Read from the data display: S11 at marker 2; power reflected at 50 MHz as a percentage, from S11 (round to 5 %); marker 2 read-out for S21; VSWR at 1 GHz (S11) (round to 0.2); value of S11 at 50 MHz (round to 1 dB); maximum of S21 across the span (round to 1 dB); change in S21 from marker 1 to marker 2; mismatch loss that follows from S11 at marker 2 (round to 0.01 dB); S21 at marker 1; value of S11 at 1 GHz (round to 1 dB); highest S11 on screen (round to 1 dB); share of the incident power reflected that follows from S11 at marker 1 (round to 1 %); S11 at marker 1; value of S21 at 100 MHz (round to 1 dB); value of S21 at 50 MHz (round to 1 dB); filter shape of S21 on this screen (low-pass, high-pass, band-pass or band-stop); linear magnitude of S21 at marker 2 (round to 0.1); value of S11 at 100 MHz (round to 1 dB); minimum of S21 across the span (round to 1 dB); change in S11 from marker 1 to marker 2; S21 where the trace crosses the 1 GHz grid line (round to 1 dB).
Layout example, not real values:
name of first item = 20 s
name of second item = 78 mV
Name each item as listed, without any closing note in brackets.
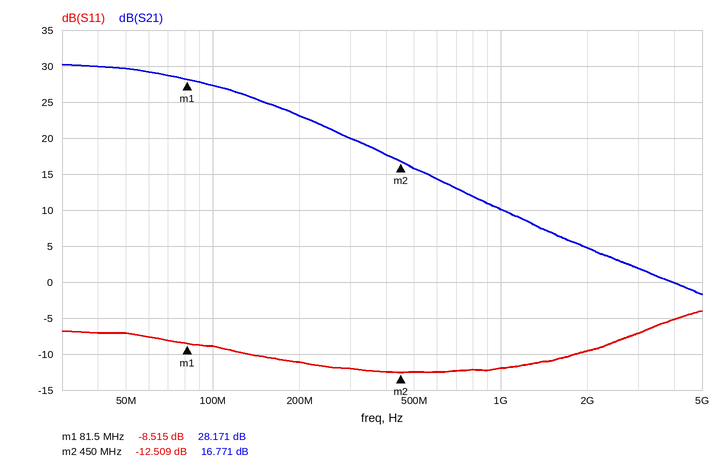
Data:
S11 at marker 2 = -12.509 dB
power reflected at 50 MHz as a percentage, from S11 = 20 %
marker 2 read-out for S21 = 16.771 dB
VSWR at 1 GHz (S11) = 1.6
value of S11 at 50 MHz = -7 dB
maximum of S21 across the span = 30 dB
change in S21 from marker 1 to marker 2 = -11.400 dB
mismatch loss that follows from S11 at marker 2 = 0.25 dB
S21 at marker 1 = 28.171 dB
value of S11 at 1 GHz = -12 dB
highest S11 on screen = -4 dB
share of the incident power reflected that follows from S11 at marker 1 = 14 %
S11 at marker 1 = -8.515 dB
value of S21 at 100 MHz = 27 dB
value of S21 at 50 MHz = 30 dB
filter shape of S21 on this screen = low-pass
linear magnitude of S21 at marker 2 = 6.9
value of S11 at 100 MHz = -9 dB
minimum of S21 across the span = -2 dB
change in S11 from marker 1 to marker 2 = -3.994 dB
S21 where the trace crosses the 1 GHz grid line = 10 dB
